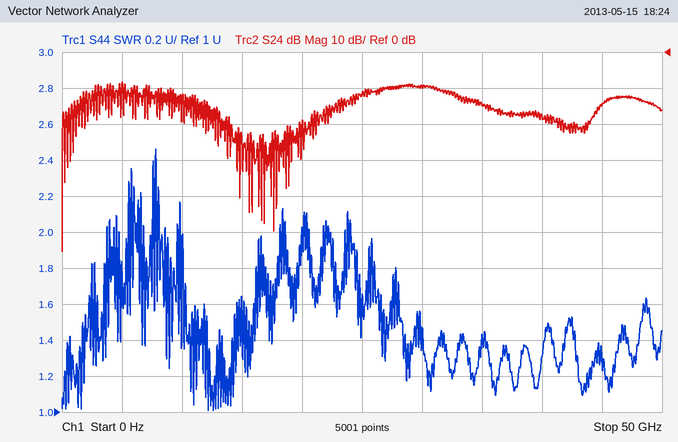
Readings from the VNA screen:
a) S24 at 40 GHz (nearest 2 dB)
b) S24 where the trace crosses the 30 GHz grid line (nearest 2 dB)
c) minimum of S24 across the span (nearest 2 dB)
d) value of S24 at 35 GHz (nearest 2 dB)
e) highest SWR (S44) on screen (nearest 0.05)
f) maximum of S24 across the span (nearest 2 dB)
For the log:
-18 dB
-10 dB
-56 dB
-14 dB
2.45
-8 dB
